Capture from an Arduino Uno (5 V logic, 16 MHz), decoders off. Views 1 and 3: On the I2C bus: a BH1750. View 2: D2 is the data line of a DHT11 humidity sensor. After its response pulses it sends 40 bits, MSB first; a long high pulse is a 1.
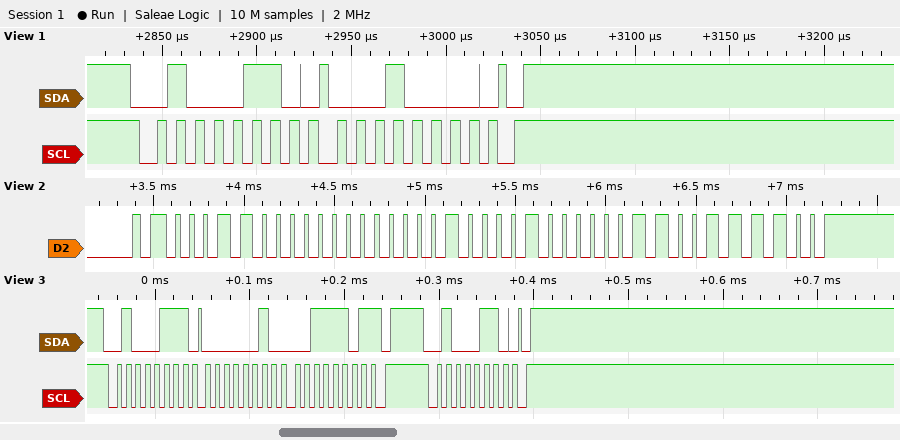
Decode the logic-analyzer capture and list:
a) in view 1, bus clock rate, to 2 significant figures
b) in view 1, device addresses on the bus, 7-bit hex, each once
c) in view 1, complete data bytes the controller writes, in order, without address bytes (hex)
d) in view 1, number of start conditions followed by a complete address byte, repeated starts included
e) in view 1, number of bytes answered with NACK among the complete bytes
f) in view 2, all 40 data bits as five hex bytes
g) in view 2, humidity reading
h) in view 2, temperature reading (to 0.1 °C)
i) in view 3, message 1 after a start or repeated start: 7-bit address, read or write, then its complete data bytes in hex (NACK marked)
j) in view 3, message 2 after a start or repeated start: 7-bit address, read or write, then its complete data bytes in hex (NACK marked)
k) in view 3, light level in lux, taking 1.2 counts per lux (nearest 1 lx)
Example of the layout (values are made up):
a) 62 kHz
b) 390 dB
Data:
a) 100 kHz
b) 0x23
c) 10
d) 1
e) 0
f) 18 00 21 03 3C
g) 24 %
h) 33.3 °C
i) 0x23 read: 02 3D NACK
j) 0x23 write
k) 478 lx
